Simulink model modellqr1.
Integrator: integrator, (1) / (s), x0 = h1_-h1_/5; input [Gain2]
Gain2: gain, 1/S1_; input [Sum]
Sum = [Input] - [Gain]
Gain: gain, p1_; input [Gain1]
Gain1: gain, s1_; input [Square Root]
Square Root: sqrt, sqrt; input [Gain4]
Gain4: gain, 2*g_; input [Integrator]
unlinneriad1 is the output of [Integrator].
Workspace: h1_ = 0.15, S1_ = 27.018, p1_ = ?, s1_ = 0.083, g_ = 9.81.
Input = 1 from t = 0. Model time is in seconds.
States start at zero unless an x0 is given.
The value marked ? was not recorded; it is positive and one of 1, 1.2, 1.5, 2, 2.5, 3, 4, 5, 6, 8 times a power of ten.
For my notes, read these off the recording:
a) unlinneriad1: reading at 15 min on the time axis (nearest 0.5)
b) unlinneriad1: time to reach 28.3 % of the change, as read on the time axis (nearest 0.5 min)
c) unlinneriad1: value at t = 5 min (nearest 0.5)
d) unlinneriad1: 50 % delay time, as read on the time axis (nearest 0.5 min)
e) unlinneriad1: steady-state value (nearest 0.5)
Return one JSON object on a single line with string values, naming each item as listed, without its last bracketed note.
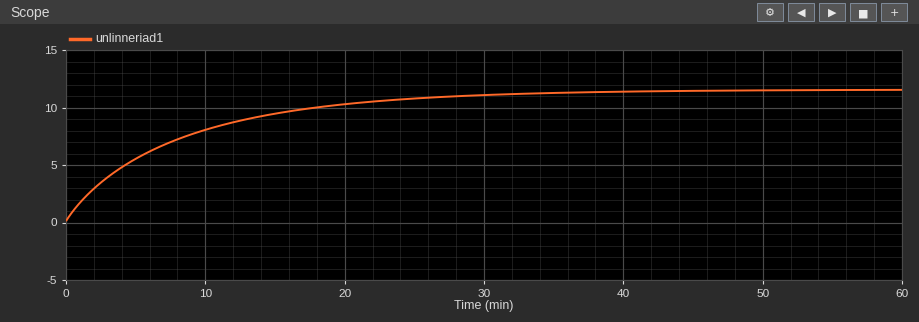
{"unlinneriad1: reading at 15 min on the time axis": "9.5", "unlinneriad1: time to reach 28.3 % of the change, as read on the time axis": "2.5 min", "unlinneriad1: value at t = 5 min": "5.5", "unlinneriad1: 50 % delay time, as read on the time axis": "5.5 min", "unlinneriad1: steady-state value": "11.5"}
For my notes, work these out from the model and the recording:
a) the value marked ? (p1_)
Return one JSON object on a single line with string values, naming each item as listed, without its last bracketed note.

{"the value marked ?": "0.8"}
